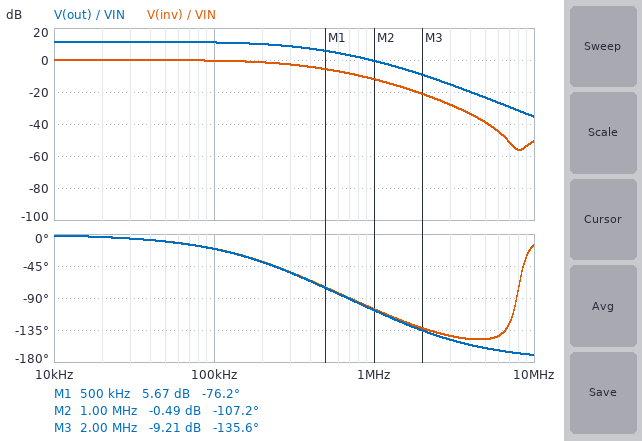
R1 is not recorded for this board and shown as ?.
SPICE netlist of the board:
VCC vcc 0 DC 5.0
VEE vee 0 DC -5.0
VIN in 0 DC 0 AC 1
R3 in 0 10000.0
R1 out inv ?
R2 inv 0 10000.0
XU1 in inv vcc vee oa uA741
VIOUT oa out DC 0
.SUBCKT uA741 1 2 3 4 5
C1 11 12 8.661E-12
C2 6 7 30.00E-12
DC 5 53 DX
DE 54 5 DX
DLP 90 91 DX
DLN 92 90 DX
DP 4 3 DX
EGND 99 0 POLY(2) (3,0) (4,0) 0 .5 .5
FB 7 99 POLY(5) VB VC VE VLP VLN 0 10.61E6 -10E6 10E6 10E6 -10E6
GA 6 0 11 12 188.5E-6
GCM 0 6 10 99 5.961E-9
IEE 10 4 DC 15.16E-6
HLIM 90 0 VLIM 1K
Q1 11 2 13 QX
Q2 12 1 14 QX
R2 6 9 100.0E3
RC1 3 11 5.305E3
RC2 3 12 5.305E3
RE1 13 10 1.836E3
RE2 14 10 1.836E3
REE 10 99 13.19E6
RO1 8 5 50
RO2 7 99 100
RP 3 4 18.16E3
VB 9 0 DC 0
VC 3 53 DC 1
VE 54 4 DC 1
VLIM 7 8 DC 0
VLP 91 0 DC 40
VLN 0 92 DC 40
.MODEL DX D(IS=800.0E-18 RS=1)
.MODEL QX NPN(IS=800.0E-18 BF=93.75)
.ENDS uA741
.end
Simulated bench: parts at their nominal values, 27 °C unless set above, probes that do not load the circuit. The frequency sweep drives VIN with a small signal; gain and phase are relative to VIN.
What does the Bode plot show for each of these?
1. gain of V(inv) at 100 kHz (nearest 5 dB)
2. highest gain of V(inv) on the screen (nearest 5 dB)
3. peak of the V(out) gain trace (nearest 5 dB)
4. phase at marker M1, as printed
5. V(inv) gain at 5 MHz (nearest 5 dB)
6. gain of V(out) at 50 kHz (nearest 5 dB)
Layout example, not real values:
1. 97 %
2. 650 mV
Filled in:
1. 0 dB
2. 0 dB
3. 10 dB
4. -76.2 deg
5. -40 dB
6. 10 dB
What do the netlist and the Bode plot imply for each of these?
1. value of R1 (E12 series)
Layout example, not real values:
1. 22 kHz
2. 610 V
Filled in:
1. 27 kΩ
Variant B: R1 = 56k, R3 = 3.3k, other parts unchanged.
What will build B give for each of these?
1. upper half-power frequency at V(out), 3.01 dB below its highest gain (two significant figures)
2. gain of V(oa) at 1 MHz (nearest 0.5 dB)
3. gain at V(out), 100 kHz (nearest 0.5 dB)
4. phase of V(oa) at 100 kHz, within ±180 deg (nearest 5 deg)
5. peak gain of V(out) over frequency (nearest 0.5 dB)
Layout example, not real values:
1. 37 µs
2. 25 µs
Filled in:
1. 160 kHz
2. -1.0 dB
3. 15.0 dB
4. -35 deg
5. 16.5 dB
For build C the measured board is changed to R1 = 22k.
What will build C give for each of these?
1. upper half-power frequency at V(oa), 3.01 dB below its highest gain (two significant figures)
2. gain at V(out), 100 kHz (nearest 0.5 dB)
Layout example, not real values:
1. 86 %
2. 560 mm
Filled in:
1. 370 kHz
2. 10.0 dB
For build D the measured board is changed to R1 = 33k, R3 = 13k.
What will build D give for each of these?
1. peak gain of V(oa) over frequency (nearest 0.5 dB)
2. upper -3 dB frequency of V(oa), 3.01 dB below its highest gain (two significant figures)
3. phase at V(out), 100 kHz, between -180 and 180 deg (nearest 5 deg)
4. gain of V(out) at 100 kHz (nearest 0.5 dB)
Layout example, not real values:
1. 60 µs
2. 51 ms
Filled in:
1. 12.5 dB
2. 260 kHz
3. -25 deg
4. 12.0 dB
